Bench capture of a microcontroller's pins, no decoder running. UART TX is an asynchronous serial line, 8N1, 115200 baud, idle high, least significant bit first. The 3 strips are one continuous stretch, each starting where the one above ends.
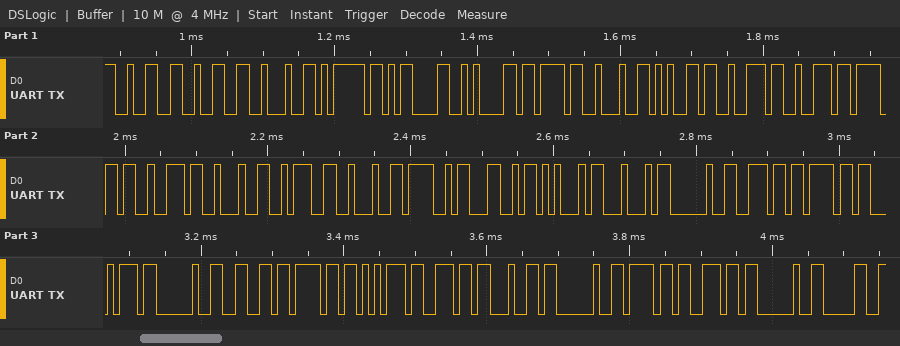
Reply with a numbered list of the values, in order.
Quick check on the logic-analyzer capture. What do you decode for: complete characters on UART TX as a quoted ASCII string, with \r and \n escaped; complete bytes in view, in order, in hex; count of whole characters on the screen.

1. "22\"}\r\n{\"error\":\"OLED not found on 0"
2. 32 32 22 7D 0D 0A 7B 22 65 72 72 6F 72 22 3A 22 4F 4C 45 44 20 6E 6F 74 20 66 6F 75 6E 64 20 6F 6E 20 30
3. 35
